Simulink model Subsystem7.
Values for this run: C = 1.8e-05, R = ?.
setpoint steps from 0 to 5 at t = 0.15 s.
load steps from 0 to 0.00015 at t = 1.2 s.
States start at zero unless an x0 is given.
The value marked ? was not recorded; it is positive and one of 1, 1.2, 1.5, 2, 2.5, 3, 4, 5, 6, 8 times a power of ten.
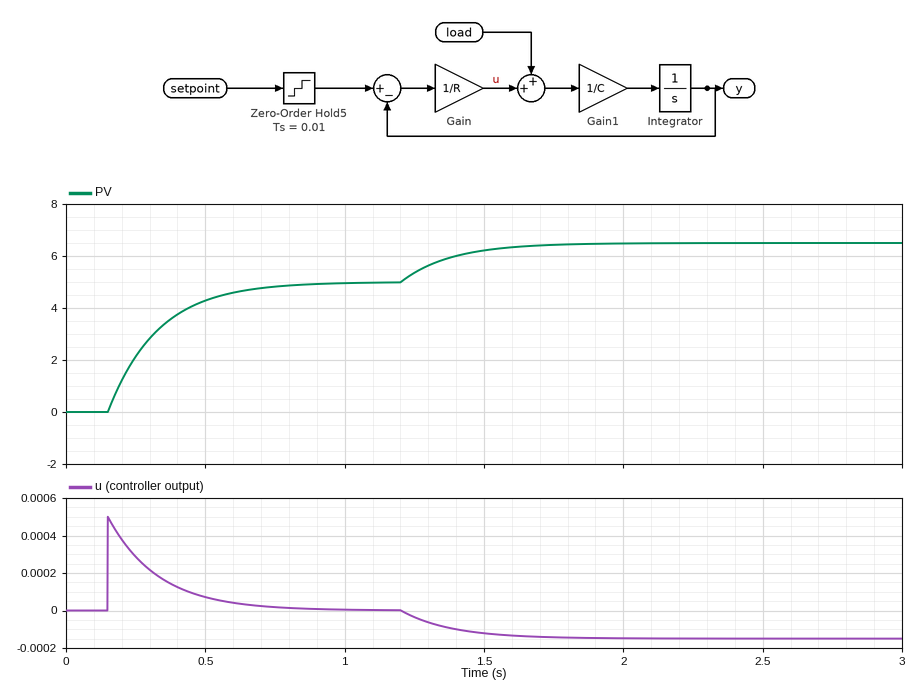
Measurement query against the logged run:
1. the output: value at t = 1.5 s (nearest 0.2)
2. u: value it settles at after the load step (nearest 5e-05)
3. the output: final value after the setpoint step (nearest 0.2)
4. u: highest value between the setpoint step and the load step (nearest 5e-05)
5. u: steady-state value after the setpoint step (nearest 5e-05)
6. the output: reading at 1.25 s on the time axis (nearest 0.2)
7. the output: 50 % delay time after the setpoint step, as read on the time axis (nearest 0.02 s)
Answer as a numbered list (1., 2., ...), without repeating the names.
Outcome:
1. 6.2
2. -0.00015
3. 5.0
4. 0.00050
5. 0.00000
6. 5.4
7. 0.28 s
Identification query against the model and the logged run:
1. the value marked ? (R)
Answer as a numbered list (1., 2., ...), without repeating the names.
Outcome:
1. 10000
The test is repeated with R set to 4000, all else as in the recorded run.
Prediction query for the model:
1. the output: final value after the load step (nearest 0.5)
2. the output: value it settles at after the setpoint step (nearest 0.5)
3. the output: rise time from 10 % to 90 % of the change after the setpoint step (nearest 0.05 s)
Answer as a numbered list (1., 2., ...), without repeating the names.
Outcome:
1. 5.5
2. 5.0
3. 0.15 s
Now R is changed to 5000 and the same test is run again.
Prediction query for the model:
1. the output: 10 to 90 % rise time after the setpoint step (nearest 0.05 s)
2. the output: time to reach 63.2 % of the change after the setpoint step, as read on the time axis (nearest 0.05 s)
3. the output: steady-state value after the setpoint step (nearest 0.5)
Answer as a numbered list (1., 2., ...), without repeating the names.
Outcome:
1. 0.20 s
2. 0.25 s
3. 5.0
